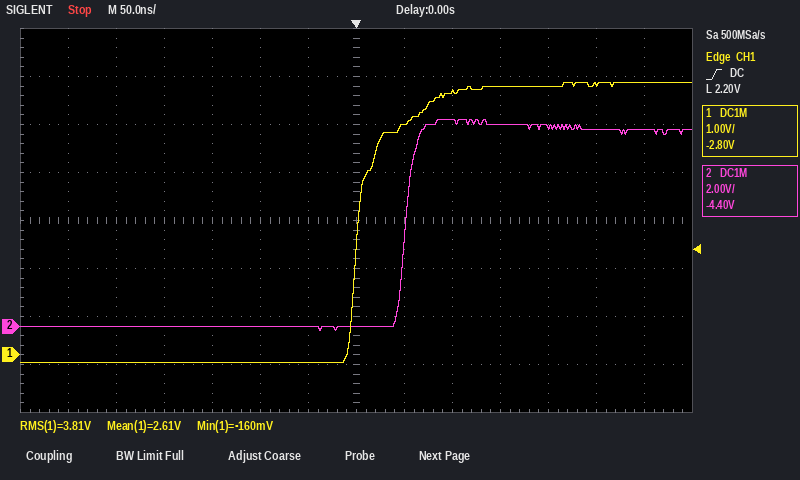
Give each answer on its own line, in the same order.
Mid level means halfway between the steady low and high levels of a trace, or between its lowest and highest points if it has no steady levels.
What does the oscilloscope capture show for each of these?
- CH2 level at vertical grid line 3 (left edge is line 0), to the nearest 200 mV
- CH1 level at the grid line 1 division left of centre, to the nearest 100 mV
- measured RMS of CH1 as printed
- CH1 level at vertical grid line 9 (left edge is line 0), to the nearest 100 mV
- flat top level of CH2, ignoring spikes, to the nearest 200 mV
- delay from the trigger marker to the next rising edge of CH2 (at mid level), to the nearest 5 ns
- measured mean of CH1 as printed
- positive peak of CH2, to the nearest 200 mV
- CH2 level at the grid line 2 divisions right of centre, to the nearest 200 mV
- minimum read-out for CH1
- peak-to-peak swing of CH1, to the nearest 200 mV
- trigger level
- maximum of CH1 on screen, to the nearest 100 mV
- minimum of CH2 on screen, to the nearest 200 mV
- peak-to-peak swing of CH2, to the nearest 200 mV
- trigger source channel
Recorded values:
0.0 V
-200 mV
3.81 V
5.5 V
8.2 V
50 ns
2.61 V
8.6 V
8.6 V
-160 mV
5.8 V
2.20 V
5.7 V
-200 mV
8.8 V
CH1
